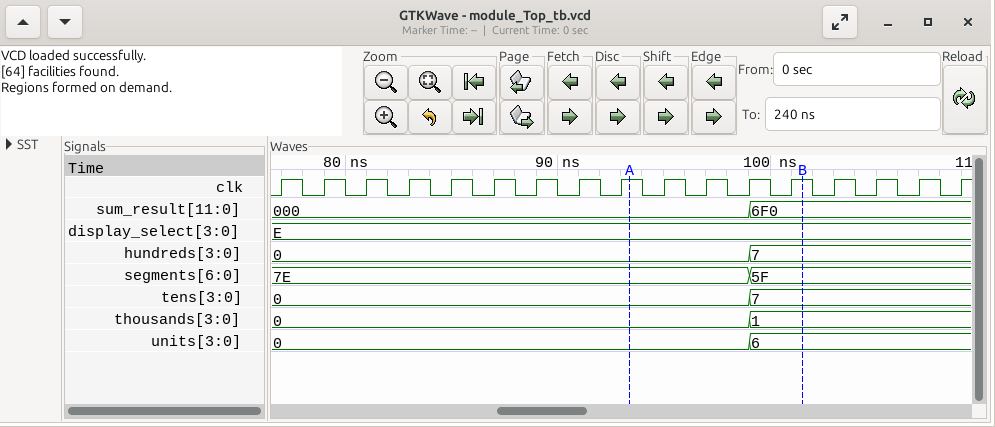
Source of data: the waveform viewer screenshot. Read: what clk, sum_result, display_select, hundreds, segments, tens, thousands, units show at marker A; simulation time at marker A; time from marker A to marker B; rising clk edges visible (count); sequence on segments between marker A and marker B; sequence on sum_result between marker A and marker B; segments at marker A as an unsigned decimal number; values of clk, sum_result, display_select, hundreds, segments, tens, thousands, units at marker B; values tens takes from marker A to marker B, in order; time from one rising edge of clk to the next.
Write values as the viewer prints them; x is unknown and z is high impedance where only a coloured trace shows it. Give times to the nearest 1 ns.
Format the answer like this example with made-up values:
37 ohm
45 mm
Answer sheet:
clk=1, sum_result=000, display_select=E, hundreds=0, segments=7E, tens=0, thousands=0, units=0
93 ns
8 ns
17
7E, 5F
000, 6F0
126
clk=1, sum_result=6F0, display_select=E, hundreds=7, segments=5F, tens=7, thousands=1, units=6
0, 7
2 ns
